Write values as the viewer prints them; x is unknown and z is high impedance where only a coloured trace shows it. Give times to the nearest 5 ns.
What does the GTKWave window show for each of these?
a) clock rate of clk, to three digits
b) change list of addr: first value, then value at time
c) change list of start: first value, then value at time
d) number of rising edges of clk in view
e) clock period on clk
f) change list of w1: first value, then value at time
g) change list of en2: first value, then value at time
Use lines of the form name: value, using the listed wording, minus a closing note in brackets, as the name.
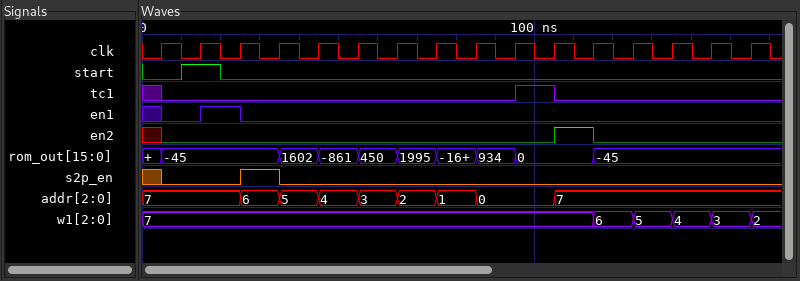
clock rate of clk, to three digits: 100 MHz
change list of addr: first value, then value at time: 7, 6 at 25 ns, 5 at 35 ns, 4 at 45 ns, 3 at 55 ns, 2 at 65 ns, 1 at 75 ns, 0 at 85 ns, 7 at 105 ns
change list of start: first value, then value at time: 0, 1 at 10 ns, 0 at 20 ns
number of rising edges of clk in view: 16
clock period on clk: 10 ns
change list of w1: first value, then value at time: 7, 6 at 115 ns, 5 at 125 ns, 4 at 135 ns, 3 at 145 ns, 2 at 155 ns
change list of en2: first value, then value at time: x, 0 at 5 ns, 1 at 105 ns, 0 at 115 ns
